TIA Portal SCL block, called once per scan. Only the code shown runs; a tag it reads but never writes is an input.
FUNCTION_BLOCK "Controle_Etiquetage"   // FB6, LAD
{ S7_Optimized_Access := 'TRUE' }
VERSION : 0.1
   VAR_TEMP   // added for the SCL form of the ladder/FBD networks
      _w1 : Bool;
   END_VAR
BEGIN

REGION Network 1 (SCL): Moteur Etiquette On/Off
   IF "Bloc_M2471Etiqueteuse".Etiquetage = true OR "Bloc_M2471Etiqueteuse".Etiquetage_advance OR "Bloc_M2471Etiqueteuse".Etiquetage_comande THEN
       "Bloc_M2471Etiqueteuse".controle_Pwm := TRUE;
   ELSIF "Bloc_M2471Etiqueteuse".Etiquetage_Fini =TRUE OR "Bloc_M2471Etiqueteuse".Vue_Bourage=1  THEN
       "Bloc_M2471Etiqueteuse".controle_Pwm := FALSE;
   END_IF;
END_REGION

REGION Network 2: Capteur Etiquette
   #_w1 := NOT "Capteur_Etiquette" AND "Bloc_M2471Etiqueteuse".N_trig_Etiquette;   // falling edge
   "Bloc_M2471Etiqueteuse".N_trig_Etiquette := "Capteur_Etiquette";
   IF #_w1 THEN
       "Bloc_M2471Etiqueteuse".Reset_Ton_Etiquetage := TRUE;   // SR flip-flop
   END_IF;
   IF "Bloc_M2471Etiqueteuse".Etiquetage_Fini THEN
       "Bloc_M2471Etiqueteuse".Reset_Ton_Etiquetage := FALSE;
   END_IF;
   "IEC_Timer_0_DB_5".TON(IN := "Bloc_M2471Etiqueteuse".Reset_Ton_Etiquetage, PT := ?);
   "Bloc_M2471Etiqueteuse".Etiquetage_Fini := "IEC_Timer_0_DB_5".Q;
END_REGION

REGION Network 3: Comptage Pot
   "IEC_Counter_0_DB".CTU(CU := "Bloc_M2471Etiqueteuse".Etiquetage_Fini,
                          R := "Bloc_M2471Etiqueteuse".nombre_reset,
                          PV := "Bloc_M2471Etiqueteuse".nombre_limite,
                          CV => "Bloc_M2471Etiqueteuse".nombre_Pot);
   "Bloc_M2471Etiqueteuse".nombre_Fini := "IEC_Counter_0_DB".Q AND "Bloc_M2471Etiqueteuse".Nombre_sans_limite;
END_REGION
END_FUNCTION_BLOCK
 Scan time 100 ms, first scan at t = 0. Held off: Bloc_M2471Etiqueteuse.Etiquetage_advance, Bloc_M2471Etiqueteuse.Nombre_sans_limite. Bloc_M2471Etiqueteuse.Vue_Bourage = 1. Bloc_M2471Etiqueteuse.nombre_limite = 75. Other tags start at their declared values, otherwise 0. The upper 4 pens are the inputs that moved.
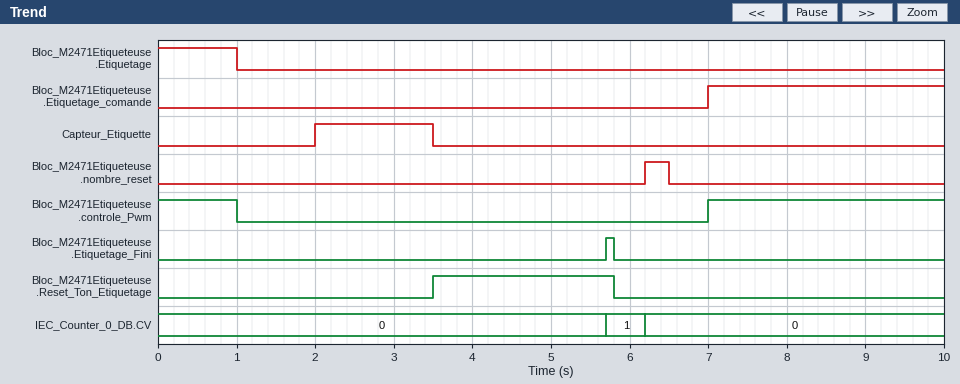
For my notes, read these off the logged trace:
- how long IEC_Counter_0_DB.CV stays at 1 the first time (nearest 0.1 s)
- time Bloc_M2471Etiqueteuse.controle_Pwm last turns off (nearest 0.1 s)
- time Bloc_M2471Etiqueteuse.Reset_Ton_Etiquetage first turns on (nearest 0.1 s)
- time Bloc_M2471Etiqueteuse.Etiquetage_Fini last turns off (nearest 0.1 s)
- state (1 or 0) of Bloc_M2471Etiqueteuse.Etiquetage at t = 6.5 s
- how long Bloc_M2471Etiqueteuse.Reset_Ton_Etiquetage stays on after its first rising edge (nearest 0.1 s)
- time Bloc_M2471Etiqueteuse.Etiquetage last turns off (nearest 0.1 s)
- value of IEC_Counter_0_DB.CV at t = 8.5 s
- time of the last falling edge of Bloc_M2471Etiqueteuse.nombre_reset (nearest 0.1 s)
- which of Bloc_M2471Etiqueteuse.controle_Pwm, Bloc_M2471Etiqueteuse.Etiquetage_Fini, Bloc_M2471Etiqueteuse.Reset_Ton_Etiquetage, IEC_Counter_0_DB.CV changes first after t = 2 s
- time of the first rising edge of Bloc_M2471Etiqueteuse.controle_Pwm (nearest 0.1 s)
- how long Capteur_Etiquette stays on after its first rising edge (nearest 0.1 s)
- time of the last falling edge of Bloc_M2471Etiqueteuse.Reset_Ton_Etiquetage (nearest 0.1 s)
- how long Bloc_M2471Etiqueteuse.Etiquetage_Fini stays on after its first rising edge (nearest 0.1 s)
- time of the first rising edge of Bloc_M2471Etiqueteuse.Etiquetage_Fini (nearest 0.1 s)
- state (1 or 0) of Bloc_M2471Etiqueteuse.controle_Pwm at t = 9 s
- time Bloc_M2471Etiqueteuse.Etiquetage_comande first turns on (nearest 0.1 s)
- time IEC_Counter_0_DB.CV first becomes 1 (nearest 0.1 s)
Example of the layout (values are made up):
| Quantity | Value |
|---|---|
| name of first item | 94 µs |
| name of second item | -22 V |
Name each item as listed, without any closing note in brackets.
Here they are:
| Quantity | Value |
|---|---|
| how long IEC_Counter_0_DB.CV stays at 1 the first time | 0.5 s |
| time Bloc_M2471Etiqueteuse.controle_Pwm last turns off | 1.0 s |
| time Bloc_M2471Etiqueteuse.Reset_Ton_Etiquetage first turns on | 3.5 s |
| time Bloc_M2471Etiqueteuse.Etiquetage_Fini last turns off | 5.8 s |
| state (1 or 0) of Bloc_M2471Etiqueteuse.Etiquetage at t = 6.5 s | 0 |
| how long Bloc_M2471Etiqueteuse.Reset_Ton_Etiquetage stays on after its first rising edge | 2.3 s |
| time Bloc_M2471Etiqueteuse.Etiquetage last turns off | 1.0 s |
| value of IEC_Counter_0_DB.CV at t = 8.5 s | 0 |
| time of the last falling edge of Bloc_M2471Etiqueteuse.nombre_reset | 6.5 s |
| which of Bloc_M2471Etiqueteuse.controle_Pwm, Bloc_M2471Etiqueteuse.Etiquetage_Fini, Bloc_M2471Etiqueteuse.Reset_Ton_Etiquetage, IEC_Counter_0_DB.CV changes first after t = 2 s | Bloc_M2471Etiqueteuse.Reset_Ton_Etiquetage |
| time of the first rising edge of Bloc_M2471Etiqueteuse.controle_Pwm | 7.0 s |
| how long Capteur_Etiquette stays on after its first rising edge | 1.5 s |
| time of the last falling edge of Bloc_M2471Etiqueteuse.Reset_Ton_Etiquetage | 5.8 s |
| how long Bloc_M2471Etiqueteuse.Etiquetage_Fini stays on after its first rising edge | 0.1 s |
| time of the first rising edge of Bloc_M2471Etiqueteuse.Etiquetage_Fini | 5.7 s |
| state (1 or 0) of Bloc_M2471Etiqueteuse.controle_Pwm at t = 9 s | 1 |
| time Bloc_M2471Etiqueteuse.Etiquetage_comande first turns on | 7.0 s |
| time IEC_Counter_0_DB.CV first becomes 1 | 5.7 s |
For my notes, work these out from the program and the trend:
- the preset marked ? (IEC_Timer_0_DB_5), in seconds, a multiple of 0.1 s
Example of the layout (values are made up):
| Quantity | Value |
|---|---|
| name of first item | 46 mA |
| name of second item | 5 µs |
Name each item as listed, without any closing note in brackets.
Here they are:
| Quantity | Value |
|---|---|
| the preset marked ? (IEC_Timer_0_DB_5), in seconds, a multiple of 0.1 s | 2.2 s |
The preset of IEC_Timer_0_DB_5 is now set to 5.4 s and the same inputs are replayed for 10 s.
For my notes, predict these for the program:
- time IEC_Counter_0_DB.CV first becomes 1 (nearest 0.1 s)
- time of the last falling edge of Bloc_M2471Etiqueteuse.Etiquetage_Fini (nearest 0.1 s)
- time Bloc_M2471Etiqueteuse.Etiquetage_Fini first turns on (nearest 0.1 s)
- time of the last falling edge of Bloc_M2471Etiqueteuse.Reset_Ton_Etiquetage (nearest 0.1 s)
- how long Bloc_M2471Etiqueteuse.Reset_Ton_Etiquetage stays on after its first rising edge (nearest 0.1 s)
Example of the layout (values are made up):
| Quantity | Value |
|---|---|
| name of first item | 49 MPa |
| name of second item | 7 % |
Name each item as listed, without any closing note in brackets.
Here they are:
| Quantity | Value |
|---|---|
| time IEC_Counter_0_DB.CV first becomes 1 | 8.9 s |
| time of the last falling edge of Bloc_M2471Etiqueteuse.Etiquetage_Fini | 9.0 s |
| time Bloc_M2471Etiqueteuse.Etiquetage_Fini first turns on | 8.9 s |
| time of the last falling edge of Bloc_M2471Etiqueteuse.Reset_Ton_Etiquetage | 9.0 s |
| how long Bloc_M2471Etiqueteuse.Reset_Ton_Etiquetage stays on after its first rising edge | 5.5 s |
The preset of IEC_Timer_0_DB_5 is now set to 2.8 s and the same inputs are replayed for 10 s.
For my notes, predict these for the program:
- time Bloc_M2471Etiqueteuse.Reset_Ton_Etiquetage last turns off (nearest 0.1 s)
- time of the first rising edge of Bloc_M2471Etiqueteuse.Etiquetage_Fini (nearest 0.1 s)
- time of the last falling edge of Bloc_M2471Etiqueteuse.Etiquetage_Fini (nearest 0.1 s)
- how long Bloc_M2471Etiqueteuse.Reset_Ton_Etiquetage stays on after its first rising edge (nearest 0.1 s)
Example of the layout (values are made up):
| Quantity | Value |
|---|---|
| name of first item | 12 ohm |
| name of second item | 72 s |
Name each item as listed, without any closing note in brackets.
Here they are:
| Quantity | Value |
|---|---|
| time Bloc_M2471Etiqueteuse.Reset_Ton_Etiquetage last turns off | 6.4 s |
| time of the first rising edge of Bloc_M2471Etiqueteuse.Etiquetage_Fini | 6.3 s |
| time of the last falling edge of Bloc_M2471Etiqueteuse.Etiquetage_Fini | 6.4 s |
| how long Bloc_M2471Etiqueteuse.Reset_Ton_Etiquetage stays on after its first rising edge | 2.9 s |
